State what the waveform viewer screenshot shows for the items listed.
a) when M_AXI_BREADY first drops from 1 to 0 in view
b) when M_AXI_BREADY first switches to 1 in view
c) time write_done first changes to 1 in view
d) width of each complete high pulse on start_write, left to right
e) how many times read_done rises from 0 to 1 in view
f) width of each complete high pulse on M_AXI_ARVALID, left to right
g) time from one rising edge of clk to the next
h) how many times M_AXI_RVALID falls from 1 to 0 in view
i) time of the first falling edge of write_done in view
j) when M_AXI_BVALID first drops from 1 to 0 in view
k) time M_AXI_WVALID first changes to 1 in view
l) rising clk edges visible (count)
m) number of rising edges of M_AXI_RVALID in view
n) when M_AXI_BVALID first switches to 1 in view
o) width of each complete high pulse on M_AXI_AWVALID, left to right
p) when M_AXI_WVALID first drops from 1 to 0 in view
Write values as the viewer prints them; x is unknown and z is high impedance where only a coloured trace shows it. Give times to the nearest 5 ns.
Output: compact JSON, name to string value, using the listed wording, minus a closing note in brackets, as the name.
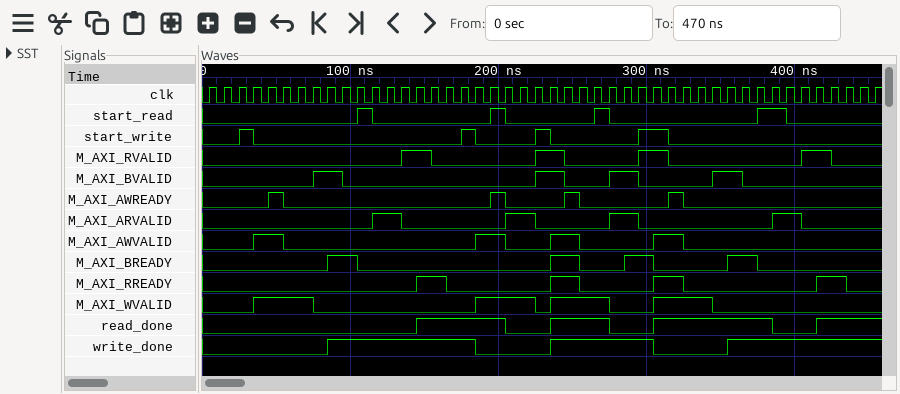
{"when M_AXI_BREADY first drops from 1 to 0 in view": "105 ns", "when M_AXI_BREADY first switches to 1 in view": "85 ns", "time write_done first changes to 1 in view": "85 ns", "width of each complete high pulse on start_write, left to right": "10 ns, 10 ns, 10 ns, 20 ns", "how many times read_done rises from 0 to 1 in view": "4", "width of each complete high pulse on M_AXI_ARVALID, left to right": "20 ns, 20 ns, 20 ns, 20 ns", "time from one rising edge of clk to the next": "10 ns", "how many times M_AXI_RVALID falls from 1 to 0 in view": "4", "time of the first falling edge of write_done in view": "185 ns", "when M_AXI_BVALID first drops from 1 to 0 in view": "95 ns", "time M_AXI_WVALID first changes to 1 in view": "35 ns", "rising clk edges visible": "46", "number of rising edges of M_AXI_RVALID in view": "4", "when M_AXI_BVALID first switches to 1 in view": "75 ns", "width of each complete high pulse on M_AXI_AWVALID, left to right": "20 ns, 20 ns, 20 ns, 20 ns", "when M_AXI_WVALID first drops from 1 to 0 in view": "75 ns"}
